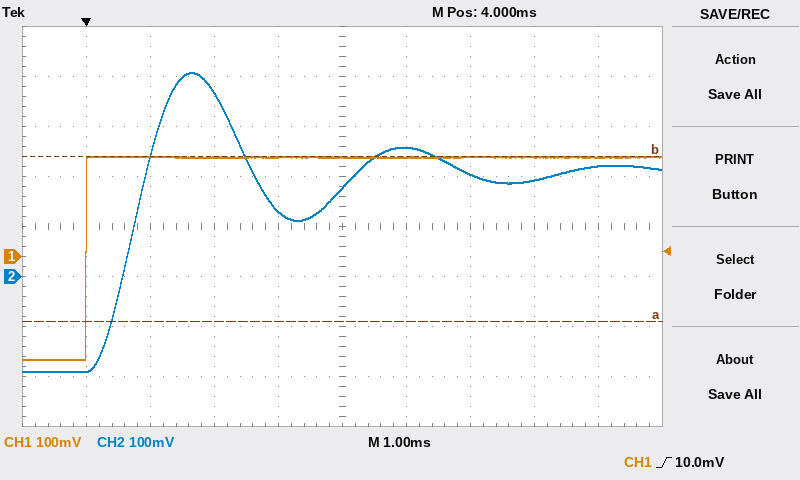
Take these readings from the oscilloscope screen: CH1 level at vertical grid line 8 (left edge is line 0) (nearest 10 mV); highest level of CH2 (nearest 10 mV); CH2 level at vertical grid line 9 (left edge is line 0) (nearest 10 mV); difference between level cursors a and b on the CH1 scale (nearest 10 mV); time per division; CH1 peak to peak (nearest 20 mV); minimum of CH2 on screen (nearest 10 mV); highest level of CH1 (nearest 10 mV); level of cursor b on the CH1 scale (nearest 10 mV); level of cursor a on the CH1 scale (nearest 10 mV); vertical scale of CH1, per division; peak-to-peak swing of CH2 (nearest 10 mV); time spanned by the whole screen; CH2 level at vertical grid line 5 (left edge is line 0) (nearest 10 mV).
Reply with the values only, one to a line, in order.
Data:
200 mV
410 mV
220 mV
330 mV
1 ms
400 mV
-190 mV
200 mV
200 mV
-130 mV
100 mV
600 mV
10 ms
180 mV
